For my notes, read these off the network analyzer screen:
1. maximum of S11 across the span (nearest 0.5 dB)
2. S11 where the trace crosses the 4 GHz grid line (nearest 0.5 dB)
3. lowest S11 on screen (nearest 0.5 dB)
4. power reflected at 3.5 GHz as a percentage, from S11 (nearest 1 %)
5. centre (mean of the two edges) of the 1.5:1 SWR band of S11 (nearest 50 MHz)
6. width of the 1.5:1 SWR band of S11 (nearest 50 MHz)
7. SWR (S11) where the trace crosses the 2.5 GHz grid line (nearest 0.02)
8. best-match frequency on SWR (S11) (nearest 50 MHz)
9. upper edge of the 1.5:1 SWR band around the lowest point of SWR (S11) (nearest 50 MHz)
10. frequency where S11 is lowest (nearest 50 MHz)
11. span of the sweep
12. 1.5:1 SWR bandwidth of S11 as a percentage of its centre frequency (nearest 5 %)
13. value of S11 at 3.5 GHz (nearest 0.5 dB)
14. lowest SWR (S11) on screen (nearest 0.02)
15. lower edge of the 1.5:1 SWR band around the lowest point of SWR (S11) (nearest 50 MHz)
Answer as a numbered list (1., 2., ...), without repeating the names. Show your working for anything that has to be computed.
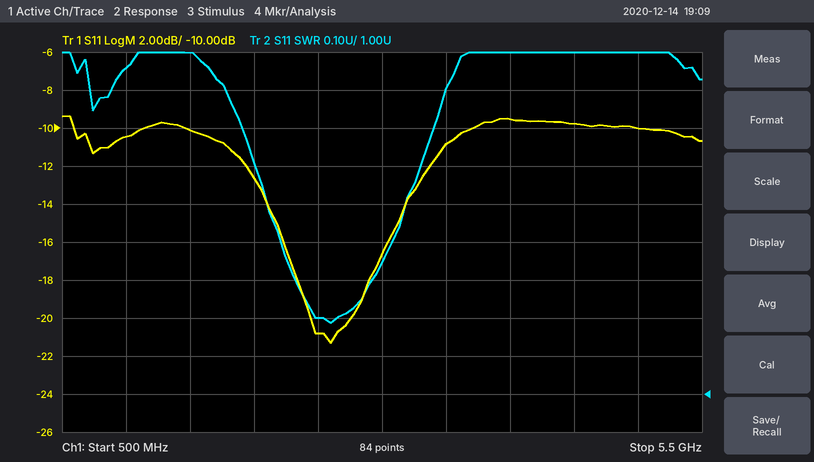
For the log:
1. -9.5 dB
2. -9.5 dB
3. -21.5 dB
4. 10^(-11/10) ≈ 8 %
5. 2.65 GHz
6. 3.20 GHz − 2.10 GHz = 1.10 GHz
7. 1.20
8. 2.60 GHz
9. 3.20 GHz
10. 2.60 GHz
11. 5 GHz
12. 1.1 GHz / 2.65 GHz ≈ 41.5 %, so 40 % to the nearest 5 %
13. -11.0 dB
14. 1.18
15. 2.10 GHz
